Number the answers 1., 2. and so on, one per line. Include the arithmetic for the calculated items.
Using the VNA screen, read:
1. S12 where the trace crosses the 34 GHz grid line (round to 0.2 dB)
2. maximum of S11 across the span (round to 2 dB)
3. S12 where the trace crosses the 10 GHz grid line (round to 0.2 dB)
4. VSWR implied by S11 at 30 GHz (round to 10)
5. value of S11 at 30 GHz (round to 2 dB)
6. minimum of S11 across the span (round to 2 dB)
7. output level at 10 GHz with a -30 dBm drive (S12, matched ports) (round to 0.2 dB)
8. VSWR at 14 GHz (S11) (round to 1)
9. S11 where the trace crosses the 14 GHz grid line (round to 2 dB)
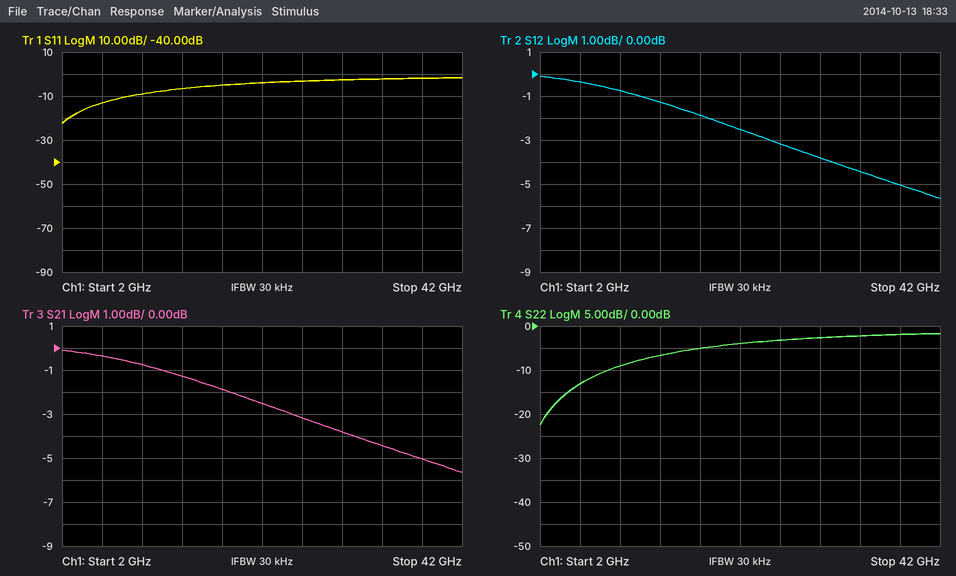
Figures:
1. -4.4 dB
2. -2 dB
3. -0.8 dB
4. |Γ| = 10^(-2/20) = 0.7943; VSWR = (1 + 0.7943)/(1 − 0.7943) ≈ 8.72, so 10 to the nearest 10
5. -2 dB
6. -22 dB
7. -30 dBm + (-0.8 dB) = -30.8 dBm
8. |Γ| = 10^(-6/20) = 0.5012; VSWR = (1 + 0.5012)/(1 − 0.5012) ≈ 3
9. -6 dB
